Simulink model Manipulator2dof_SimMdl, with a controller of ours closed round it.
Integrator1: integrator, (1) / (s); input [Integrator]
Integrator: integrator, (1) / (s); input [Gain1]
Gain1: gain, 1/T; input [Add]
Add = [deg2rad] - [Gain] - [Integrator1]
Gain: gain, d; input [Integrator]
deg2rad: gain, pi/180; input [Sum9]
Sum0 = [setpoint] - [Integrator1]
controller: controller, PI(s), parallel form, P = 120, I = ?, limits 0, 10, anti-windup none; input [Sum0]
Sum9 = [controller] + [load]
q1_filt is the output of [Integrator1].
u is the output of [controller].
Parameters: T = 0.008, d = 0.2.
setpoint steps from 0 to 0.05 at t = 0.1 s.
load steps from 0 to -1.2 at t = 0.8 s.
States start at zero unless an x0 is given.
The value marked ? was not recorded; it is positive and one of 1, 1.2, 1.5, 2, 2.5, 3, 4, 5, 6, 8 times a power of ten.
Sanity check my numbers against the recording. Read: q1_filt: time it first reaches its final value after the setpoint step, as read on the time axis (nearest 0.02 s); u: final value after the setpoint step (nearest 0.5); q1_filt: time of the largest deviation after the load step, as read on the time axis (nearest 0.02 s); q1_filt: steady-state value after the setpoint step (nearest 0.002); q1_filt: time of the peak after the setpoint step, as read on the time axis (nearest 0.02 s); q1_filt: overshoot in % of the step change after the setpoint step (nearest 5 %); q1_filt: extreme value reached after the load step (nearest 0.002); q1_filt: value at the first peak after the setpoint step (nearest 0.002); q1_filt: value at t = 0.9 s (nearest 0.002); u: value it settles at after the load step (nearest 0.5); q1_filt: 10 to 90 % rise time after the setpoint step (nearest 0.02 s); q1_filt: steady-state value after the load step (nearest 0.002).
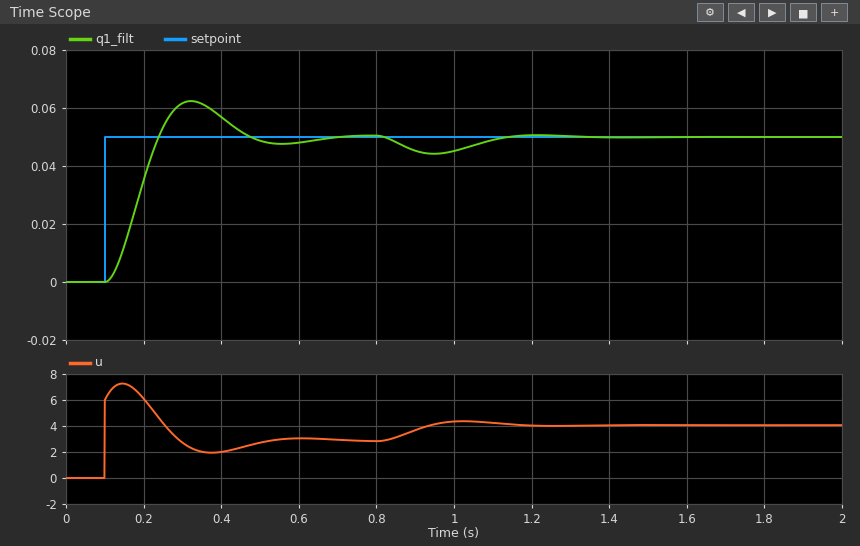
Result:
0.24 s
3.0
0.94 s
0.050
0.32 s
25 %
0.044
0.062
0.046
4.0
0.10 s
0.050
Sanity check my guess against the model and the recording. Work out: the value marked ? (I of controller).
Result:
1200
